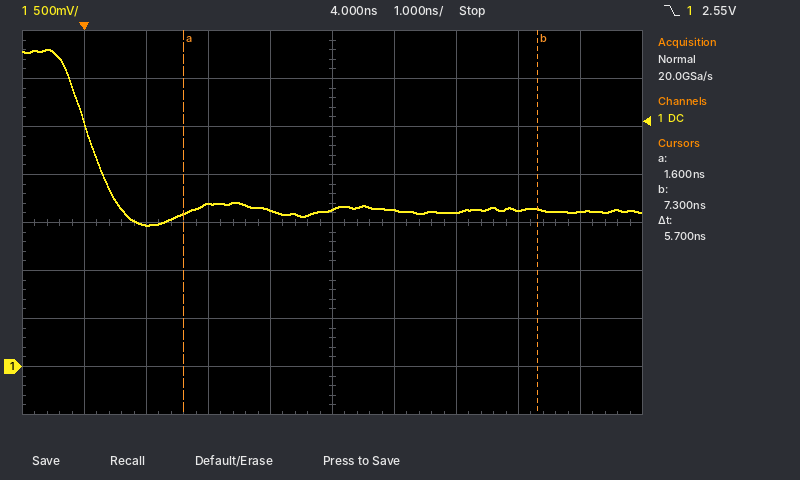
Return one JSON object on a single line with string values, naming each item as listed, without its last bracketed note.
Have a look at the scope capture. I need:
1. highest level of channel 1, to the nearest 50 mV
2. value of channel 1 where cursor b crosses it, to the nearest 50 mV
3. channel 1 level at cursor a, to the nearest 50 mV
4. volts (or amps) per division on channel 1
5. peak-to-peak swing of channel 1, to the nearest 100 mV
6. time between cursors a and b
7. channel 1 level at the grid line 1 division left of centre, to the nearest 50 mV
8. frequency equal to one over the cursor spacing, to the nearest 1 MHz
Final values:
{"highest level of channel 1, to the nearest 50 mV": "3.30 V", "value of channel 1 where cursor b crosses it, to the nearest 50 mV": "1.65 V", "channel 1 level at cursor a, to the nearest 50 mV": "1.60 V", "volts (or amps) per division on channel 1": "500 mV", "peak-to-peak swing of channel 1, to the nearest 100 mV": "1.80 V", "time between cursors a and b": "5.7 ns", "channel 1 level at the grid line 1 division left of centre, to the nearest 50 mV": "1.65 V", "frequency equal to one over the cursor spacing, to the nearest 1 MHz": "175 MHz"}
